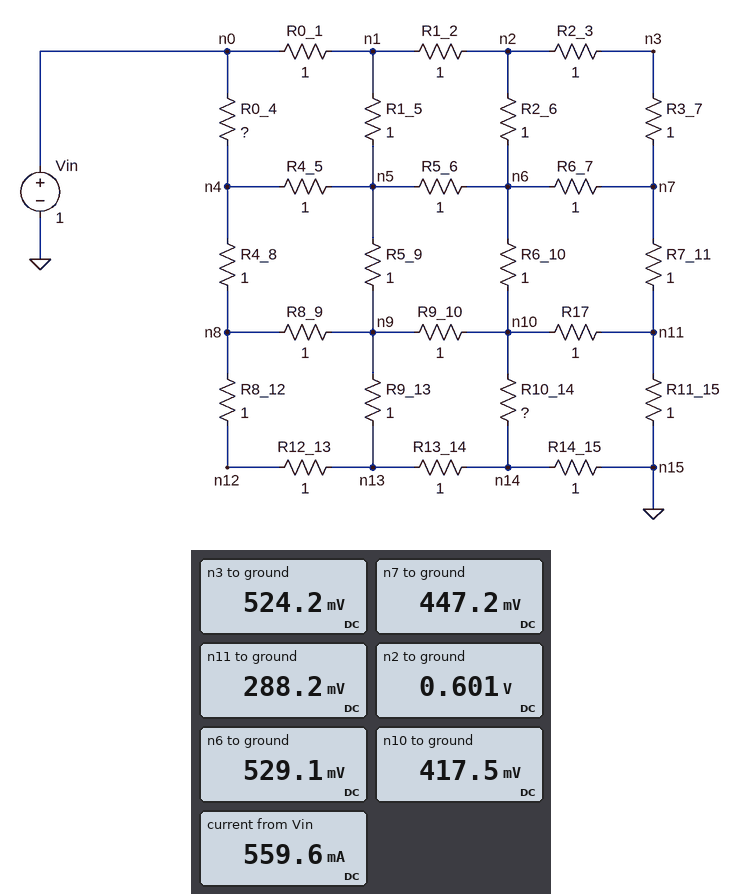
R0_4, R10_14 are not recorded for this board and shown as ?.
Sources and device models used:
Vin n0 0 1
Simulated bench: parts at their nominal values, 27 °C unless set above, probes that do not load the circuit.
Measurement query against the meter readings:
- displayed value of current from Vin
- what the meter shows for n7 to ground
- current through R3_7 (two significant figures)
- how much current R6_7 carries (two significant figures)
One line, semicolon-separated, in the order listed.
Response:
559.6 mA; 447.2 mV; 77 mA; 82 mA
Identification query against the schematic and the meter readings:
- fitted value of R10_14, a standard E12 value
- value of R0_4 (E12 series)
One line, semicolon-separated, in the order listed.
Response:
1.5 Ω; 0.68 Ω
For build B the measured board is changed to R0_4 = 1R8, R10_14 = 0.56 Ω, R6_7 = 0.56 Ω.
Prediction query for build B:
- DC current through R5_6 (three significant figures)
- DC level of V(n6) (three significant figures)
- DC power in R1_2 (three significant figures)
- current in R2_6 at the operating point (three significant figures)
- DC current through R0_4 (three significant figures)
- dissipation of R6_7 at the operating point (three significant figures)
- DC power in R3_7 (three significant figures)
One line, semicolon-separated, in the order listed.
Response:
109 mA; 448 mV; 25.5 mW; 90.5 mA; 203 mA; 4.13 mW; 4.80 mW
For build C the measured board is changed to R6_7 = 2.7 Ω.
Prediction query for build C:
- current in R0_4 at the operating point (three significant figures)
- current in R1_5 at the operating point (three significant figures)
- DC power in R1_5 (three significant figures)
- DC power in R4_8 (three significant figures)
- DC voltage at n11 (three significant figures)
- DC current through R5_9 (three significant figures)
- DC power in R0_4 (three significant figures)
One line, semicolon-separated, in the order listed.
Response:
306 mA; 96.6 mA; 9.33 mW; 29.2 mW; 280 mV; 120 mA; 63.7 mW
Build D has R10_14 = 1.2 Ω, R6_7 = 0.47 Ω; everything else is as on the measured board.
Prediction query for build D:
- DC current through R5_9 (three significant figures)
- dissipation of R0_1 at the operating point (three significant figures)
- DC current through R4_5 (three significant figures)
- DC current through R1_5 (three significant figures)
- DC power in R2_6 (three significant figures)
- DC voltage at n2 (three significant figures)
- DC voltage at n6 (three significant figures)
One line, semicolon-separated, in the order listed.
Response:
116 mA; 64.0 mW; 143 mA; 103 mA; 6.92 mW; 597 mV; 514 mV
